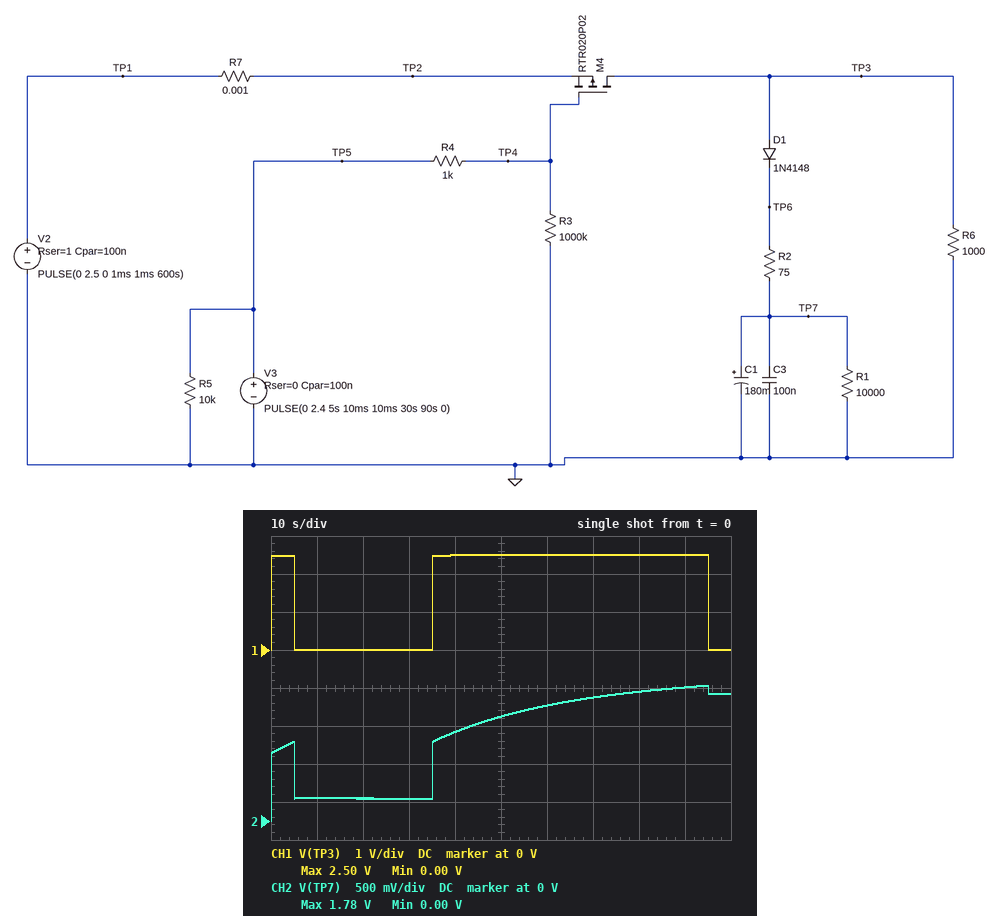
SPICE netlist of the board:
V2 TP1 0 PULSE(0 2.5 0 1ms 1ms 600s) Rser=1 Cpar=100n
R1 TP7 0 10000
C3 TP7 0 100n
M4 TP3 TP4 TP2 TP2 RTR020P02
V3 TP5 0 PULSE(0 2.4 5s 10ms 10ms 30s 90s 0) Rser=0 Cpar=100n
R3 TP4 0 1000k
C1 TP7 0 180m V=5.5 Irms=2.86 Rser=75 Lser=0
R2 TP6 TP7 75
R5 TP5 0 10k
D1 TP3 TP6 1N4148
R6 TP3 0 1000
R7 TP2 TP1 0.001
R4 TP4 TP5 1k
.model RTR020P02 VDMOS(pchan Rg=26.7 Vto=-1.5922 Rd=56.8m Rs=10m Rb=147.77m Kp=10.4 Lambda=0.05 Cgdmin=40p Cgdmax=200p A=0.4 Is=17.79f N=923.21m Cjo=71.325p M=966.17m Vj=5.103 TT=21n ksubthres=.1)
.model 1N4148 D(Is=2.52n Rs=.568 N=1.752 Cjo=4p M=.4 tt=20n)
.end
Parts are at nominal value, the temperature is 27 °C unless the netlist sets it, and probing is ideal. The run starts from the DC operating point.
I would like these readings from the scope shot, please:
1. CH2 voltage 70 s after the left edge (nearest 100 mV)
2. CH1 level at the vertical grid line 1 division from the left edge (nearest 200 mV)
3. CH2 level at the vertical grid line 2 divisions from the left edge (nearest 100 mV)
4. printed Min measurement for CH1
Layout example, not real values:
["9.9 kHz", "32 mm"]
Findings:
["1.6 V", "0 V", "300 mV", "0.00 V"]
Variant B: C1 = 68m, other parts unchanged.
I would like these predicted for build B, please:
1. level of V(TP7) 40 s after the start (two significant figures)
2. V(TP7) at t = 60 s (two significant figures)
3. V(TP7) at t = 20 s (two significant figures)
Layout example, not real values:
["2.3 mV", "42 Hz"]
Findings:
["1.5 V", "1.8 V", "670 mV"]
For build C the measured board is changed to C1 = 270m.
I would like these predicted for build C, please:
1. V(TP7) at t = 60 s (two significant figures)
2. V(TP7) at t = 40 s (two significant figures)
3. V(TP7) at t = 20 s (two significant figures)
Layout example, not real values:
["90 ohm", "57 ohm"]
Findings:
["1.4 V", "1.1 V", "200 mV"]
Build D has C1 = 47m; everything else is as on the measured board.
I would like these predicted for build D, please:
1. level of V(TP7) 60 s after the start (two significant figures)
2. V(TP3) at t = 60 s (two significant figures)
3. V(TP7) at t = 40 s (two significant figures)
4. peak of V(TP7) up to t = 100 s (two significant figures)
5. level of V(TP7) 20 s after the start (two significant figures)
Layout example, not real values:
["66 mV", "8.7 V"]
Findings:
["1.9 V", "2.5 V", "1.6 V", "2.0 V", "880 mV"]
